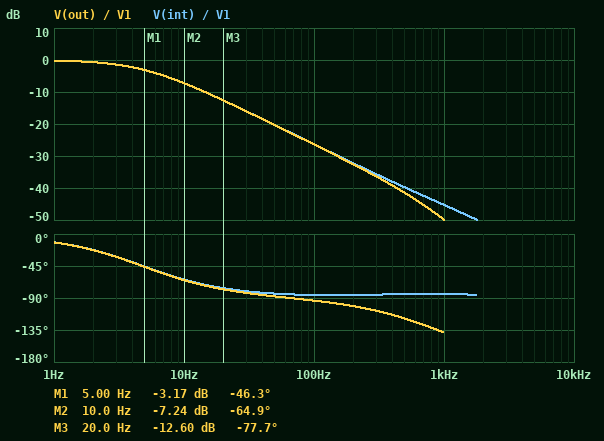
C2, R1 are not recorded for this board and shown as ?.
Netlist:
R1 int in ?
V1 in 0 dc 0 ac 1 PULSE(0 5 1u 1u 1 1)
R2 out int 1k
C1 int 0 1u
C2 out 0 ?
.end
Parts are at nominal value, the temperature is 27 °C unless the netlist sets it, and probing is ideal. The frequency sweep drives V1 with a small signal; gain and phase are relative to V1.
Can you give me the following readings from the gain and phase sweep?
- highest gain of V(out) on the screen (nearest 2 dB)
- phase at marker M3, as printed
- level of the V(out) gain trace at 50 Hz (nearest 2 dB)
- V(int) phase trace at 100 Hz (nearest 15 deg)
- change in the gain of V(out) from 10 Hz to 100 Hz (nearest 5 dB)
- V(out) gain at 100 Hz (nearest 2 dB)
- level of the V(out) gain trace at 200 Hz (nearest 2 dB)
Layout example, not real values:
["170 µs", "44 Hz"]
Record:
["0 dB", "-77.7 deg", "-20 dB", "-90 deg", "-20 dB", "-26 dB", "-32 dB"]
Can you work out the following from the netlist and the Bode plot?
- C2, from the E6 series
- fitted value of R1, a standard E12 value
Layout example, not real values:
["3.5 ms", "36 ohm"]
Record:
["220 nF", "27 kΩ"]
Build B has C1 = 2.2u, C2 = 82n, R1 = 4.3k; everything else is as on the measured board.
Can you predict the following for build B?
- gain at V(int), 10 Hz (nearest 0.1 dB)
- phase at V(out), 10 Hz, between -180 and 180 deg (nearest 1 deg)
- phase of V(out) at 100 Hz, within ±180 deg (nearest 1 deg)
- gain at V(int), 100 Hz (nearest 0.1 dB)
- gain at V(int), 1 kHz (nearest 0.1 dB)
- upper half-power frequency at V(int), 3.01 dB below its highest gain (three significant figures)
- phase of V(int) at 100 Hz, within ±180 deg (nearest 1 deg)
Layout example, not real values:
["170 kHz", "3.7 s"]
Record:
["-1.4 dB", "-32 deg", "-84 deg", "-15.9 dB", "-35.7 dB", "16.2 Hz", "-81 deg"]
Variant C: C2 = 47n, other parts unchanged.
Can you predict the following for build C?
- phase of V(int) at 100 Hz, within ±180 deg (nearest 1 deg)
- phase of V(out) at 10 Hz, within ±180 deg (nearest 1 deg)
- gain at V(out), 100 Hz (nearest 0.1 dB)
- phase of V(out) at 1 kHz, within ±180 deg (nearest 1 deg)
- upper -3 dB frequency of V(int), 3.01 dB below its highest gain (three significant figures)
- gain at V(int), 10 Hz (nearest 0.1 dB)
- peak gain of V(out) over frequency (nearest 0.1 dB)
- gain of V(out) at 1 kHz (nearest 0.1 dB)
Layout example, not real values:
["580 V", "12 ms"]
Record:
["-87 deg", "-61 deg", "-25.0 dB", "-105 deg", "5.63 Hz", "-6.2 dB", "0 dB", "-45.3 dB"]
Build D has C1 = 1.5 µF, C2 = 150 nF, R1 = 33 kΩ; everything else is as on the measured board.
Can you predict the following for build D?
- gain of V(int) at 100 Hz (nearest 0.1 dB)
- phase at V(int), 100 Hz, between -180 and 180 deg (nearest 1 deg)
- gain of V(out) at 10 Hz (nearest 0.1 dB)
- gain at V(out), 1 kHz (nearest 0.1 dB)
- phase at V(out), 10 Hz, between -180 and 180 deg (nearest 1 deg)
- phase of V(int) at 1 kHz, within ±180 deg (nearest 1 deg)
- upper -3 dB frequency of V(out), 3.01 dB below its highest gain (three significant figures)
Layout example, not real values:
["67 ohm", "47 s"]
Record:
["-30.7 dB", "-88 deg", "-11.0 dB", "-53.1 dB", "-74 deg", "-87 deg", "2.92 Hz"]
